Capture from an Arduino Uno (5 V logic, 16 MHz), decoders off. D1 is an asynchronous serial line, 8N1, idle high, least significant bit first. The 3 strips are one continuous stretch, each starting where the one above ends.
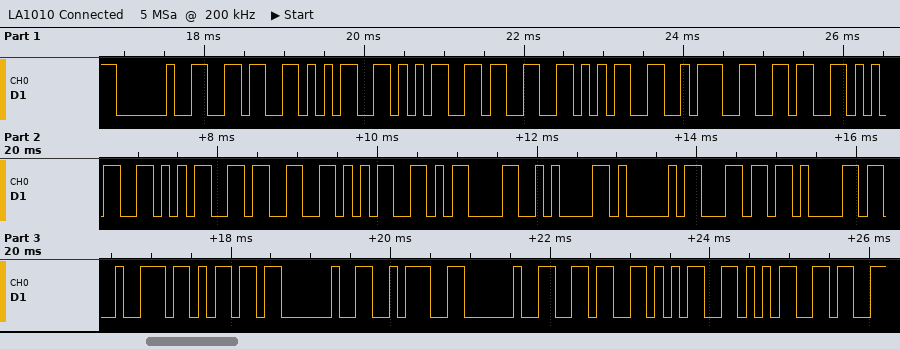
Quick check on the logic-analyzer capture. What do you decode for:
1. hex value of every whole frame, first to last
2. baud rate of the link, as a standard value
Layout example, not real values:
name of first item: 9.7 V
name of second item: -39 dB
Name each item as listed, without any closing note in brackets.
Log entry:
hex value of every whole frame, first to last: 20 36 35 35 33 35 3A 36 35 35 33 35 0D 0A 41 6C 61 72 6D 20 3A 20 36 35 35
baud rate of the link, as a standard value: 9600 baud
